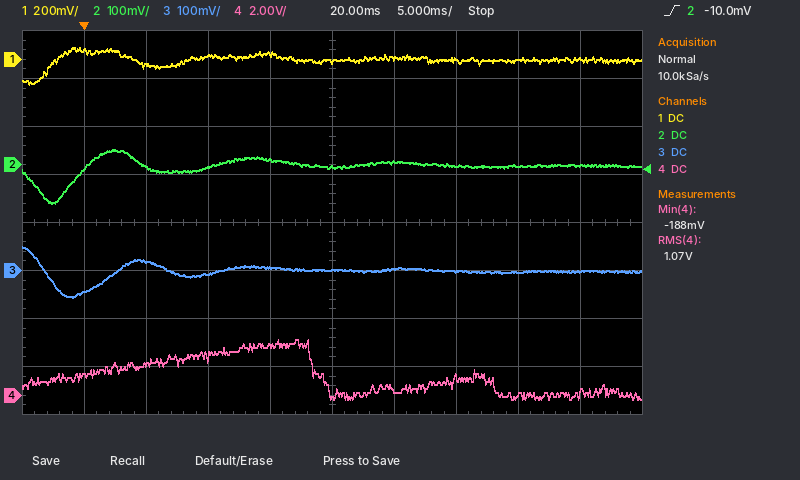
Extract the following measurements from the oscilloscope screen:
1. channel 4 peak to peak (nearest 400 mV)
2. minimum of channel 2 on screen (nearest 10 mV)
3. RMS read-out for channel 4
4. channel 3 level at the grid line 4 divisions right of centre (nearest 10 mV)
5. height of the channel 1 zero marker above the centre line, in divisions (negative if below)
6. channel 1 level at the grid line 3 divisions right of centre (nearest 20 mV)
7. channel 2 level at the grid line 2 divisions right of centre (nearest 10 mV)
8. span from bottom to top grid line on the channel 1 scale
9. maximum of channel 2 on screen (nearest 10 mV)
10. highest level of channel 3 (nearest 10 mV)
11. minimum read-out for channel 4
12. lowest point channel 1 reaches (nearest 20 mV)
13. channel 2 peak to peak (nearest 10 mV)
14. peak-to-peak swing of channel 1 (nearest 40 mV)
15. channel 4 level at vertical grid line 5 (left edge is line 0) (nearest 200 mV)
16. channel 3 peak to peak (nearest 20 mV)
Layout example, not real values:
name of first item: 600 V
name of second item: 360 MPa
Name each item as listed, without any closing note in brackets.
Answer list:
channel 4 peak to peak: 2.4 V
minimum of channel 2 on screen: -80 mV
RMS read-out for channel 4: 1.07 V
channel 3 level at the grid line 4 divisions right of centre: 0 mV
height of the channel 1 zero marker above the centre line, in divisions: +3.4 div
channel 1 level at the grid line 3 divisions right of centre: 0 mV
channel 2 level at the grid line 2 divisions right of centre: 0 mV
span from bottom to top grid line on the channel 1 scale: 1.6 V
maximum of channel 2 on screen: 30 mV
highest level of channel 3: 50 mV
minimum read-out for channel 4: -188 mV
lowest point channel 1 reaches: -100 mV
channel 2 peak to peak: 110 mV
peak-to-peak swing of channel 1: 160 mV
channel 4 level at vertical grid line 5 (left edge is line 0): 0.0 V
channel 3 peak to peak: 100 mV
